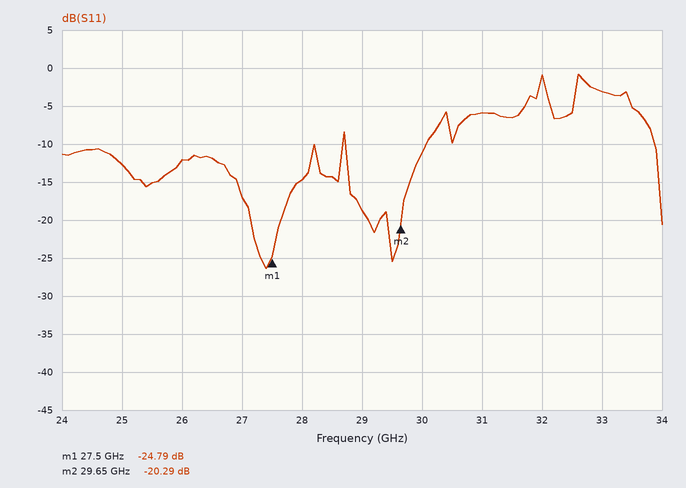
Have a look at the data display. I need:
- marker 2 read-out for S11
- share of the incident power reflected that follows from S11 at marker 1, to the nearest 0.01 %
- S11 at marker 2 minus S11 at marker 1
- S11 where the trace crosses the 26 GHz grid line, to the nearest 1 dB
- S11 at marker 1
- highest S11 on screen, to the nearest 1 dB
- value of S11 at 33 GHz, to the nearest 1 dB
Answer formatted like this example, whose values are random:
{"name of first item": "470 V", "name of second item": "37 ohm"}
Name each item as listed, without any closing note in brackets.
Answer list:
{"marker 2 read-out for S11": "-20.29 dB", "share of the incident power reflected that follows from S11 at marker 1, to the nearest 0.01 %": "0.33 %", "S11 at marker 2 minus S11 at marker 1": "4.50 dB", "S11 where the trace crosses the 26 GHz grid line, to the nearest 1 dB": "-12 dB", "S11 at marker 1": "-24.79 dB", "highest S11 on screen, to the nearest 1 dB": "-1 dB", "value of S11 at 33 GHz, to the nearest 1 dB": "-3 dB"}
